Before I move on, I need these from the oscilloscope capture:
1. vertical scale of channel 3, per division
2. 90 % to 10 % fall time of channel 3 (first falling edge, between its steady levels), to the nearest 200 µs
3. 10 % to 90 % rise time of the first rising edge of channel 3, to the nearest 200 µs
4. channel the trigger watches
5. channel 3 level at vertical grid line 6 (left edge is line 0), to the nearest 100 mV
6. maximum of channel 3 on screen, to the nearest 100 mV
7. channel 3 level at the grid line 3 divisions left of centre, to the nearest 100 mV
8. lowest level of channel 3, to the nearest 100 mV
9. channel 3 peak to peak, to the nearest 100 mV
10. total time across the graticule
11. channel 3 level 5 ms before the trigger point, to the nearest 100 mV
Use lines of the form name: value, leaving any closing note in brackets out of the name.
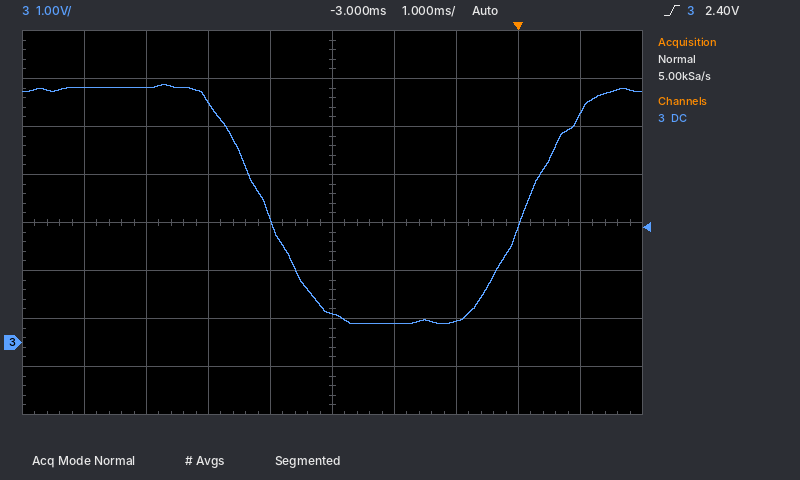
vertical scale of channel 3, per division: 1 V
90 % to 10 % fall time of channel 3 (first falling edge, between its steady levels), to the nearest 200 µs: 1.6 ms
10 % to 90 % rise time of the first rising edge of channel 3, to the nearest 200 µs: 1.6 ms
channel the trigger watches: channel 3
channel 3 level at vertical grid line 6 (left edge is line 0), to the nearest 100 mV: 400 mV
maximum of channel 3 on screen, to the nearest 100 mV: 5.4 V
channel 3 level at the grid line 3 divisions left of centre, to the nearest 100 mV: 5.3 V
lowest level of channel 3, to the nearest 100 mV: 400 mV
channel 3 peak to peak, to the nearest 100 mV: 5.0 V
total time across the graticule: 10 ms
channel 3 level 5 ms before the trigger point, to the nearest 100 mV: 5.0 V
